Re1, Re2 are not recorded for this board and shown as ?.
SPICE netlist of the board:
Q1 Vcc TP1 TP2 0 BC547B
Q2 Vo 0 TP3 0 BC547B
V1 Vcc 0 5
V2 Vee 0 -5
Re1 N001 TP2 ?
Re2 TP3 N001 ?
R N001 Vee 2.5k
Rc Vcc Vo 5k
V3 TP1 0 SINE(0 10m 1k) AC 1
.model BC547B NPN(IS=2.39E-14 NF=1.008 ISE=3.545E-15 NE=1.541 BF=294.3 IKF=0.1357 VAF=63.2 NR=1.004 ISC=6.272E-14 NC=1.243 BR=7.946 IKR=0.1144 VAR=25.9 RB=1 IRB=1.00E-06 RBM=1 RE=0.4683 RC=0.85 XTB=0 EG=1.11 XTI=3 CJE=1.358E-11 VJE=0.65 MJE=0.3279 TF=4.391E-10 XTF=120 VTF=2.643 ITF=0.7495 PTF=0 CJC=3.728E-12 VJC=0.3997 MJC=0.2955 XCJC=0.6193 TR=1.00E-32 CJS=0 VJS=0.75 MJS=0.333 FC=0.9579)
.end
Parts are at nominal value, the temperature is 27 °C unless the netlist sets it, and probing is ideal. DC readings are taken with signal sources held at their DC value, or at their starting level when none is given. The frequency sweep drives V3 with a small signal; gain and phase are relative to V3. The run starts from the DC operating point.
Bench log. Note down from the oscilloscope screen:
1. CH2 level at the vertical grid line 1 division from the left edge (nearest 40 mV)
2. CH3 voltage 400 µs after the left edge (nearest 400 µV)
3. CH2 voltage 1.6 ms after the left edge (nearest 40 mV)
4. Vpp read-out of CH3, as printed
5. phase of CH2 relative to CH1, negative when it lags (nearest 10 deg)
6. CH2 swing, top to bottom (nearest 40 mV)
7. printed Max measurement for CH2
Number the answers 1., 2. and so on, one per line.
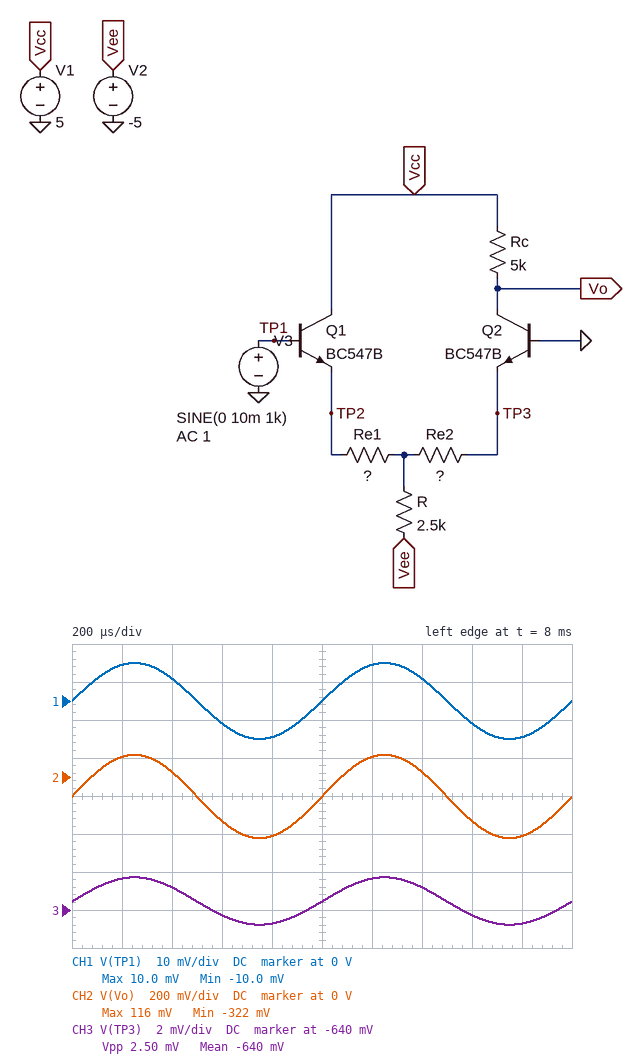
1. 120 mV
2. -638.8 mV
3. -240 mV
4. 2.50 mV
5. 0 deg
6. 440 mV
7. 116 mV
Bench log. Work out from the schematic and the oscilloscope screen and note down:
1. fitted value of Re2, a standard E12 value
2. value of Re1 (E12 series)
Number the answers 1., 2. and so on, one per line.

1. 56 Ω
2. 100 Ω
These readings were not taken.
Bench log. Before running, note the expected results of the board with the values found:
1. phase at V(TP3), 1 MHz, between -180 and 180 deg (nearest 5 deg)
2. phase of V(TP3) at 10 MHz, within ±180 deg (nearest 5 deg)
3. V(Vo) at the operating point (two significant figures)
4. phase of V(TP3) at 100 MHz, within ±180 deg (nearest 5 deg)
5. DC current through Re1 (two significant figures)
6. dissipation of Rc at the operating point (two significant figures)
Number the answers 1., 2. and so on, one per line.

1. 0 deg
2. -5 deg
3. -100 mV
4. -35 deg
5. 700 µA
6. 5.2 mW
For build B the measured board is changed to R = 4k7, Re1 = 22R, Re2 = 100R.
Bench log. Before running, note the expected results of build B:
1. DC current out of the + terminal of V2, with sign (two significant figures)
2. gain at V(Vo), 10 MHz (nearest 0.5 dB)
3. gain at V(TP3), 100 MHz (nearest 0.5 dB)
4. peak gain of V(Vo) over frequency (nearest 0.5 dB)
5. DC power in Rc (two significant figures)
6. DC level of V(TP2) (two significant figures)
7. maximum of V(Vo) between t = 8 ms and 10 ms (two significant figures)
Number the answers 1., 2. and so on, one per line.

1. -930 µA
2. 24.5 dB
3. -13.0 dB
4. 26.0 dB
5. 480 µW
6. -620 mV
7. 3.6 V
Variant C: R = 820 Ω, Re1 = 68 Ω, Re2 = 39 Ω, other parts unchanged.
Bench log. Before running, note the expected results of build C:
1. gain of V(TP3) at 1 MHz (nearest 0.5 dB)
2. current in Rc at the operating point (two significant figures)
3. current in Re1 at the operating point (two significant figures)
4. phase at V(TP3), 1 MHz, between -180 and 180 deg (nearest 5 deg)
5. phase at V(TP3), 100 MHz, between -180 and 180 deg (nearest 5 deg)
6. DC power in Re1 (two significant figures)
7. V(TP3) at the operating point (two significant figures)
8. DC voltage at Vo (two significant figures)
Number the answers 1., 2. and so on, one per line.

1. -18.5 dB
2. 1.1 mA
3. 2.3 mA
4. 0 deg
5. -55 deg
6. 370 µW
7. -710 mV
8. -700 mV
